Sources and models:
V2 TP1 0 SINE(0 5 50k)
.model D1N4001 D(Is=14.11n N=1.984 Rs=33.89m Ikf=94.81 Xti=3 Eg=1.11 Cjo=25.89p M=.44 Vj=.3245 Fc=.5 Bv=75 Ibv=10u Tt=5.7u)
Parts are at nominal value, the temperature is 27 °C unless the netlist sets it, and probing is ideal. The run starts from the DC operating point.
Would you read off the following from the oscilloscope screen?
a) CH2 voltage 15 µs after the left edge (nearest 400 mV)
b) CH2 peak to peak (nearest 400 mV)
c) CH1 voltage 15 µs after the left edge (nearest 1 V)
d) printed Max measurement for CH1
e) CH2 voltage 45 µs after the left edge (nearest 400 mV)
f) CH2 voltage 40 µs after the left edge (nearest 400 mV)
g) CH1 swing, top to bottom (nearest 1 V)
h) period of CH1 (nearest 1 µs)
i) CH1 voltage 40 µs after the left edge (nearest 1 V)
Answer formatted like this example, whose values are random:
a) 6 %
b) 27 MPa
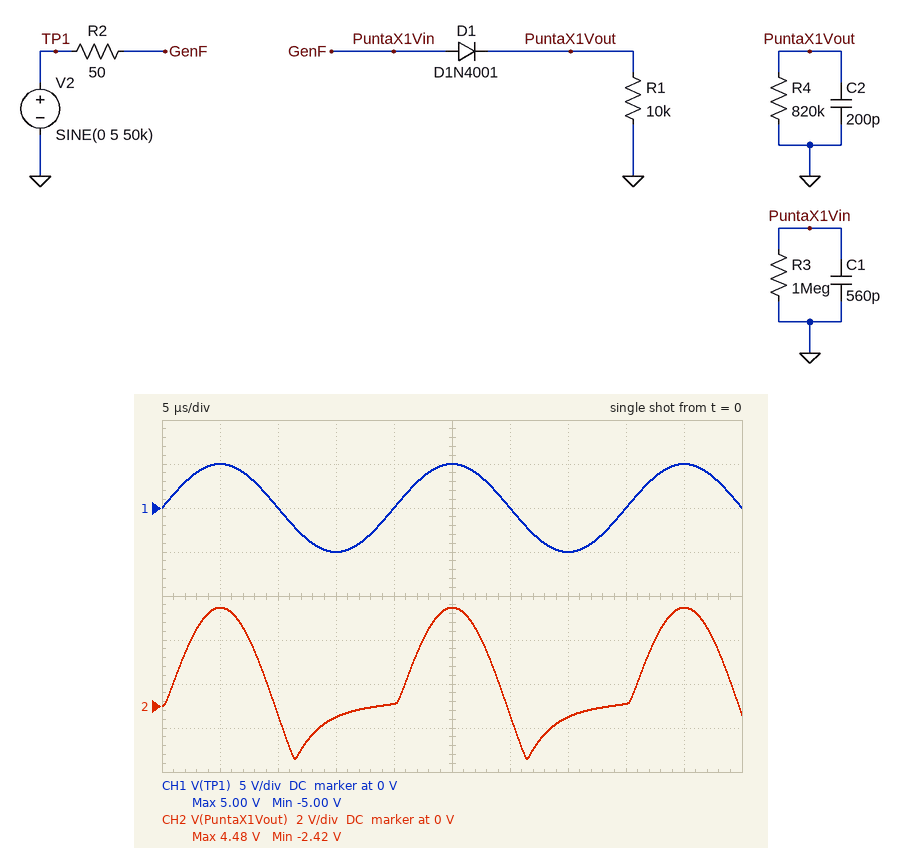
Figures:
a) -400 mV
b) 6.8 V
c) -5 V
d) 5.00 V
e) 4.4 V
f) 0 V
g) 10 V
h) 20 µs
i) 0 V
